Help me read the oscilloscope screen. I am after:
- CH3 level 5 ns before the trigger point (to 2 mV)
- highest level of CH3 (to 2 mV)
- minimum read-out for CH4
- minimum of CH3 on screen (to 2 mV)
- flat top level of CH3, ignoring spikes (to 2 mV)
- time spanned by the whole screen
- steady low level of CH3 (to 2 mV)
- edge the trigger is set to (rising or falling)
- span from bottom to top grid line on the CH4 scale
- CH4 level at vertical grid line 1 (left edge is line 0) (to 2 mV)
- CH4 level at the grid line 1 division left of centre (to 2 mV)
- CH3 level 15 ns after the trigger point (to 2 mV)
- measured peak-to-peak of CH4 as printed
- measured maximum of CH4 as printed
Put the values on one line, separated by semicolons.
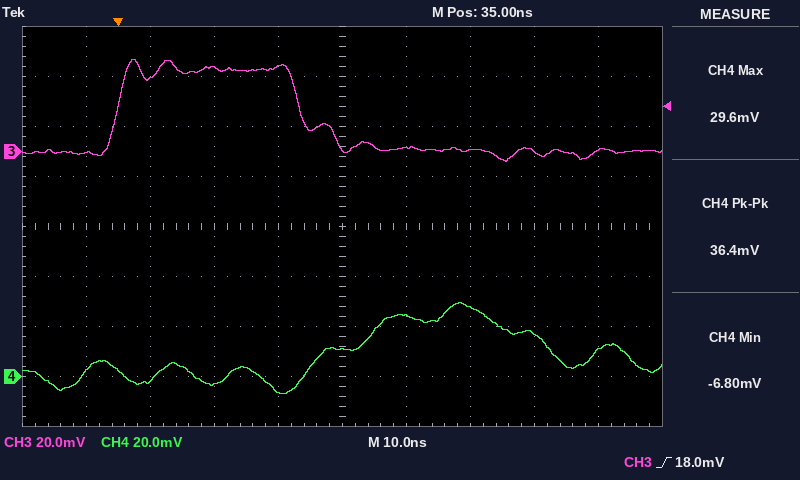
0 mV; 36 mV; -6.80 mV; -4 mV; 32 mV; 100 ns; 0 mV; rising; 160 mV; 2 mV; -6 mV; 34 mV; 36.4 mV; 29.6 mV
